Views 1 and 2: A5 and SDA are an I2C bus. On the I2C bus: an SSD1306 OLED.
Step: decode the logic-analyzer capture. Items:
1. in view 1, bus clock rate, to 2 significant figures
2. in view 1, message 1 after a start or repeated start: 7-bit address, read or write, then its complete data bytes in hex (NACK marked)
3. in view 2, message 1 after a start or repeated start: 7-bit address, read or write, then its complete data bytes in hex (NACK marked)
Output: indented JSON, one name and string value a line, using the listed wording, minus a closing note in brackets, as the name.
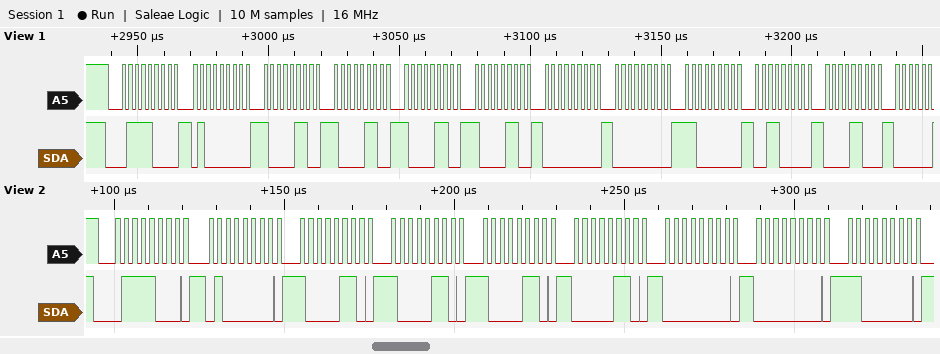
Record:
{
  "in view 1, bus clock rate, to 2 significant figures": "400 kHz",
  "in view 1, message 1 after a start or repeated start: 7-bit address, read or write, then its complete data bytes in hex": "0x3C write: 40 86 86 86 86 00 00 C0 30 0C",
  "in view 2, message 1 after a start or repeated start: 7-bit address, read or write, then its complete data bytes in hex": "0x3C write: 40 86 86 86 06 00 00 C0"
}
